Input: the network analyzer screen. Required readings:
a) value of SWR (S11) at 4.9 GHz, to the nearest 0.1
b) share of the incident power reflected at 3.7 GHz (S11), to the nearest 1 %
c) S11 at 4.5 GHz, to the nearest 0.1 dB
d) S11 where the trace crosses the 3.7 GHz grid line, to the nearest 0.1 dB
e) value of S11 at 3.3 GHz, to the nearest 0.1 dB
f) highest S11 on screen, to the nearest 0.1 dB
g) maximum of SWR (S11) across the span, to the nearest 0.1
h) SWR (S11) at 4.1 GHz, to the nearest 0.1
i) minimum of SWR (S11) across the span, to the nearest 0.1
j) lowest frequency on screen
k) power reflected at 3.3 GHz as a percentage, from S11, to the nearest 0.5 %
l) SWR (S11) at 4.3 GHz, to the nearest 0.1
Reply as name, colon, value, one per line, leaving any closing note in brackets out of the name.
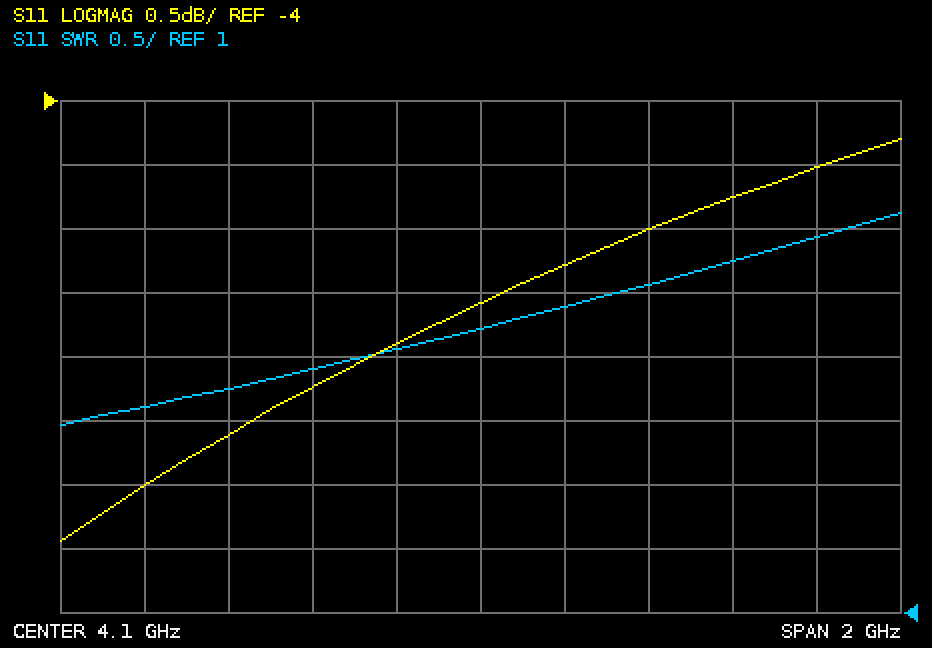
value of SWR (S11) at 4.9 GHz, to the nearest 0.1: 3.9
share of the incident power reflected at 3.7 GHz (S11), to the nearest 1 %: 24 %
S11 at 4.5 GHz, to the nearest 0.1 dB: -5.0 dB
S11 where the trace crosses the 3.7 GHz grid line, to the nearest 0.1 dB: -6.2 dB
value of S11 at 3.3 GHz, to the nearest 0.1 dB: -7.0 dB
highest S11 on screen, to the nearest 0.1 dB: -4.3 dB
maximum of SWR (S11) across the span, to the nearest 0.1: 4.1
SWR (S11) at 4.1 GHz, to the nearest 0.1: 3.2
minimum of SWR (S11) across the span, to the nearest 0.1: 2.5
lowest frequency on screen: 3.1 GHz
power reflected at 3.3 GHz as a percentage, from S11, to the nearest 0.5 %: 20.0 %
SWR (S11) at 4.3 GHz, to the nearest 0.1: 3.4
